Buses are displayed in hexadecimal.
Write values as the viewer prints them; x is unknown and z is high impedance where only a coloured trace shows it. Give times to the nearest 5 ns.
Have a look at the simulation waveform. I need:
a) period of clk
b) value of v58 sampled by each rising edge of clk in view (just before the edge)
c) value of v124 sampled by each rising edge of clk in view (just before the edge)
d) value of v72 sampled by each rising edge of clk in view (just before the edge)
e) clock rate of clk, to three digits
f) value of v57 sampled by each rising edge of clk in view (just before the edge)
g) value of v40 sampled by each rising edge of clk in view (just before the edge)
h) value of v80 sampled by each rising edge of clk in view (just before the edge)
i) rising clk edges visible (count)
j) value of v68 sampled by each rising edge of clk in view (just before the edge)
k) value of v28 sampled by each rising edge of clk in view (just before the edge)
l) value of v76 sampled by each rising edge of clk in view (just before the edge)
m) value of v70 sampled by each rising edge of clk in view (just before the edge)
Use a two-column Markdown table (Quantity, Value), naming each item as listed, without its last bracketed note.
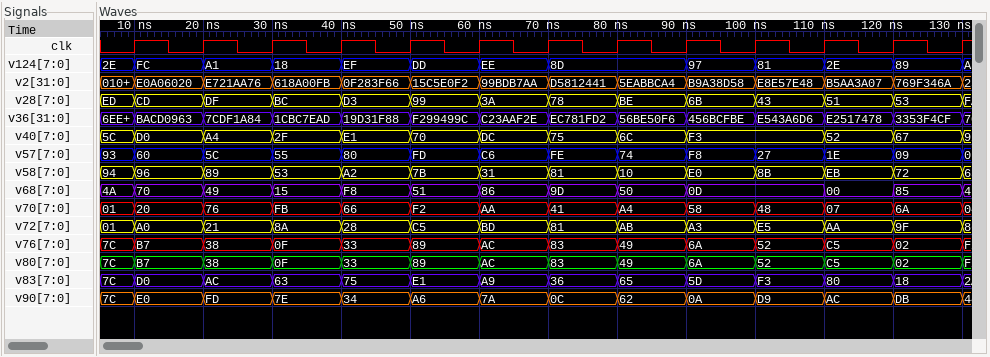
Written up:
| Quantity | Value |
|---|---|
| period of clk | 10 ns |
| value of v58 sampled by each rising edge of clk in view | 94, 96, 89, 53, A2, 7B, 31, 81, 10, E0, 8B, EB, 72 |
| value of v124 sampled by each rising edge of clk in view | 2E, FC, A1, 18, EF, DD, EE, 8D, 8D, 97, 81, 2E, 89 |
| value of v72 sampled by each rising edge of clk in view | 01, A0, 21, 8A, 28, C5, BD, 81, AB, A3, E5, AA, 9F |
| clock rate of clk, to three digits | 100 MHz |
| value of v57 sampled by each rising edge of clk in view | 93, 60, 5C, 55, 80, FD, C6, FE, 74, F8, 27, 1E, 09 |
| value of v40 sampled by each rising edge of clk in view | 5C, D0, A4, 2F, E1, 70, DC, 75, 6C, F3, F3, 52, 67 |
| value of v80 sampled by each rising edge of clk in view | 7C, B7, 38, 0F, 33, 89, AC, 83, 49, 6A, 52, C5, 02 |
| rising clk edges visible | 13 |
| value of v68 sampled by each rising edge of clk in view | 4A, 70, 49, 15, F8, 51, 86, 9D, 50, 0D, 0D, 00, 85 |
| value of v28 sampled by each rising edge of clk in view | ED, CD, DF, BC, D3, 99, 3A, 78, BE, 6B, 43, 51, 53 |
| value of v76 sampled by each rising edge of clk in view | 7C, B7, 38, 0F, 33, 89, AC, 83, 49, 6A, 52, C5, 02 |
| value of v70 sampled by each rising edge of clk in view | 01, 20, 76, FB, 66, F2, AA, 41, A4, 58, 48, 07, 6A |
